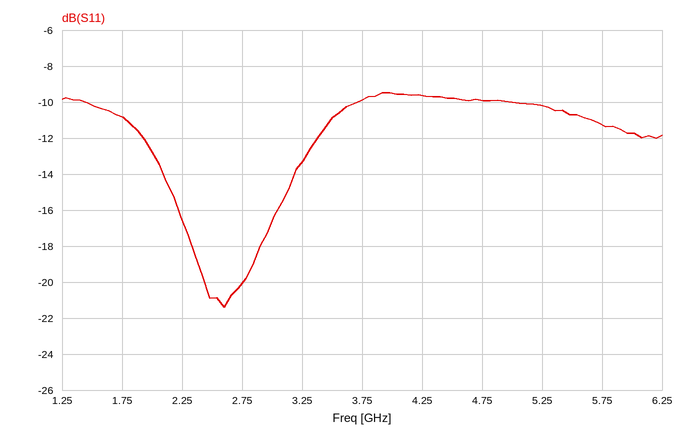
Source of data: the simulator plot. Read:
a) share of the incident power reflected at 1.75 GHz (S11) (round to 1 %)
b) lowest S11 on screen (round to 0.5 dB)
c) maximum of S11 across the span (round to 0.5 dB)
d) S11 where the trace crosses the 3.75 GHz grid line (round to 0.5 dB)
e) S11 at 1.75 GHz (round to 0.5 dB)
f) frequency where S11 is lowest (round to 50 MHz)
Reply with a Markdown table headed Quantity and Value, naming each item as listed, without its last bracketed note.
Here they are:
| Quantity | Value |
|---|---|
| share of the incident power reflected at 1.75 GHz (S11) | 8 % |
| lowest S11 on screen | -21.5 dB |
| maximum of S11 across the span | -9.5 dB |
| S11 where the trace crosses the 3.75 GHz grid line | -10.0 dB |
| S11 at 1.75 GHz | -11.0 dB |
| frequency where S11 is lowest | 2.60 GHz |
